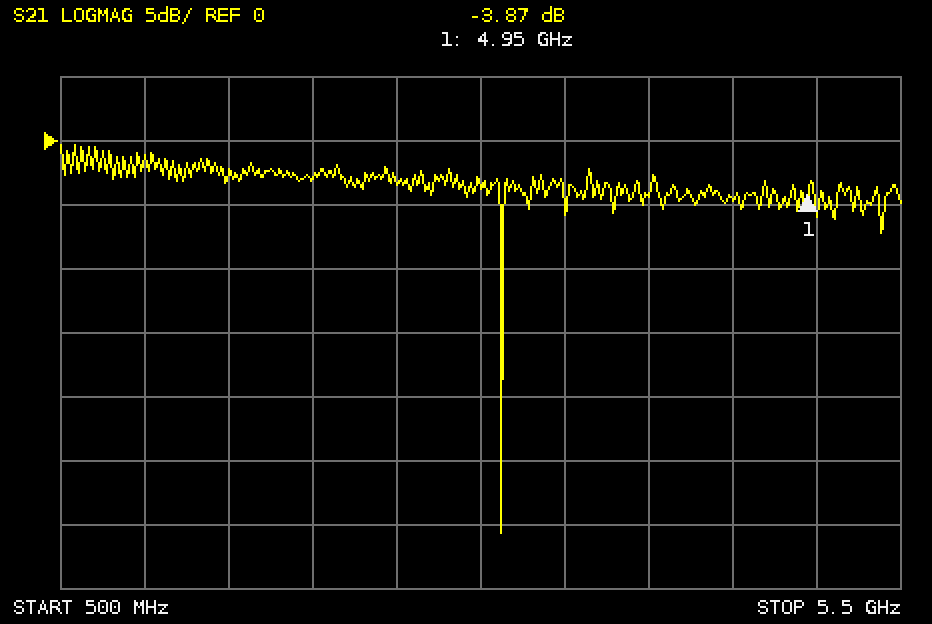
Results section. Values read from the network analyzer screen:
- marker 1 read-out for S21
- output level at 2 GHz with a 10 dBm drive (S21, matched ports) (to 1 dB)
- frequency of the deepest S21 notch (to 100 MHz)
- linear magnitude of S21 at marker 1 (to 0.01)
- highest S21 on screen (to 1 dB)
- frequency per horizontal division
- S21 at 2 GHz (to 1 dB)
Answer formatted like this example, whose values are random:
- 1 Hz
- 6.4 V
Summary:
- -3.87 dB
- 7 dBm
- 3.1 GHz
- 0.64
- 0 dB
- 500 MHz
- -3 dB
